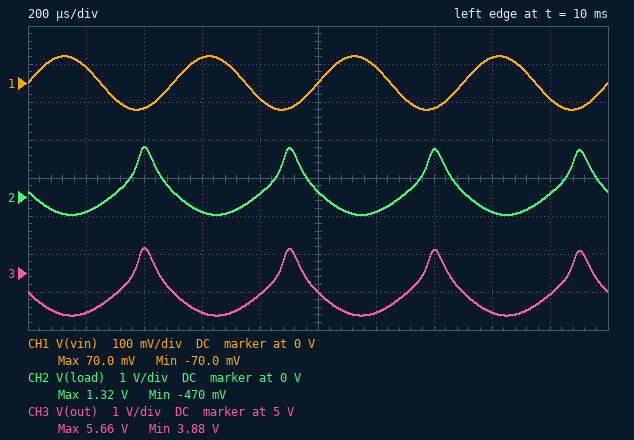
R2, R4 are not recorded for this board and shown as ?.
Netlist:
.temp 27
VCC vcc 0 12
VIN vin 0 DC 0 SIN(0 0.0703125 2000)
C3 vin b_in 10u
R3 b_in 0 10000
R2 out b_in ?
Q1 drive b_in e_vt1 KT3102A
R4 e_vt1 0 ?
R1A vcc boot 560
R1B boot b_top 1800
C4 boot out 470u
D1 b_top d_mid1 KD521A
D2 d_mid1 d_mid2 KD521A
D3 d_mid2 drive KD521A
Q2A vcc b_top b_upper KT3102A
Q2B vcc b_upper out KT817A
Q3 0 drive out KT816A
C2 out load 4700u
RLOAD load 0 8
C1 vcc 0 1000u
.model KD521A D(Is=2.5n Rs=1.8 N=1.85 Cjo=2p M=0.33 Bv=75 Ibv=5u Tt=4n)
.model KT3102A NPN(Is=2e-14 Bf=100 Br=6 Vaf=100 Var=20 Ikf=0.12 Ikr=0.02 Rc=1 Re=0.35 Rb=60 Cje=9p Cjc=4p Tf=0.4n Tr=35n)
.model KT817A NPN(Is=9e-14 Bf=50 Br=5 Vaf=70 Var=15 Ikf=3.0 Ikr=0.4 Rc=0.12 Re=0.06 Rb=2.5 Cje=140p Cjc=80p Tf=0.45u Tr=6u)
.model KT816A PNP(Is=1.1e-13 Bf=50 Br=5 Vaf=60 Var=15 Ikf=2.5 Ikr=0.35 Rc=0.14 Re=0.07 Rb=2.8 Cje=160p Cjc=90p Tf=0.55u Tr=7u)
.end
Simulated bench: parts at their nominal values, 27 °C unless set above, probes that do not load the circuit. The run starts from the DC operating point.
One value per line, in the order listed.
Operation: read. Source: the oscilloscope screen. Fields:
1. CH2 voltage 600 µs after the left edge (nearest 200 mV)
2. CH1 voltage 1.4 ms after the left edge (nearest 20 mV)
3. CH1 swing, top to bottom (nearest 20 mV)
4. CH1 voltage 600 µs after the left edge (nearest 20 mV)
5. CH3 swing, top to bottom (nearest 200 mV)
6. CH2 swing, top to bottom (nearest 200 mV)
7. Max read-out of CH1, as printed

-400 mV
-60 mV
140 mV
60 mV
1.8 V
1.8 V
70.0 mV
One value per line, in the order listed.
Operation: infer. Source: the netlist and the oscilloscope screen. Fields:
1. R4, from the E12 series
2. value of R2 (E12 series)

68 Ω
27 kΩ
